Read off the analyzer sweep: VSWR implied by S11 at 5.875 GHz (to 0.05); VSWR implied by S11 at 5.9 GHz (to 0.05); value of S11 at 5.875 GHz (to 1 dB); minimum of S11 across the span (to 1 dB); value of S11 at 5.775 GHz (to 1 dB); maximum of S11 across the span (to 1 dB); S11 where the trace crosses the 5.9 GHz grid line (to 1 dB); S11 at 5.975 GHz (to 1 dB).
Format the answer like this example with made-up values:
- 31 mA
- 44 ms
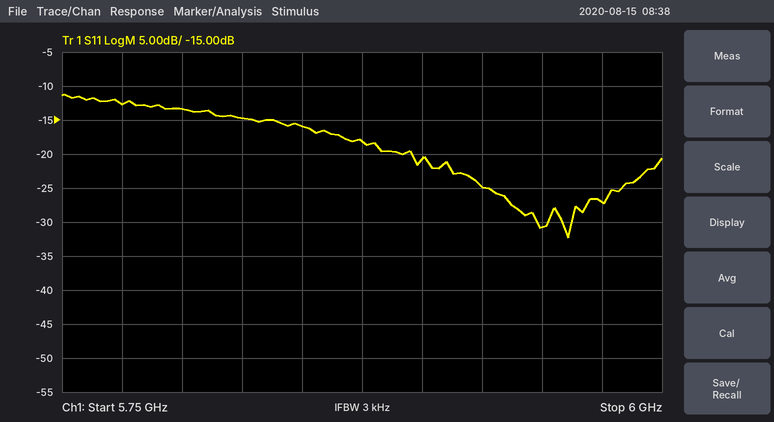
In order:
- 1.30
- 1.20
- -18 dB
- -32 dB
- -13 dB
- -11 dB
- -21 dB
- -27 dB
